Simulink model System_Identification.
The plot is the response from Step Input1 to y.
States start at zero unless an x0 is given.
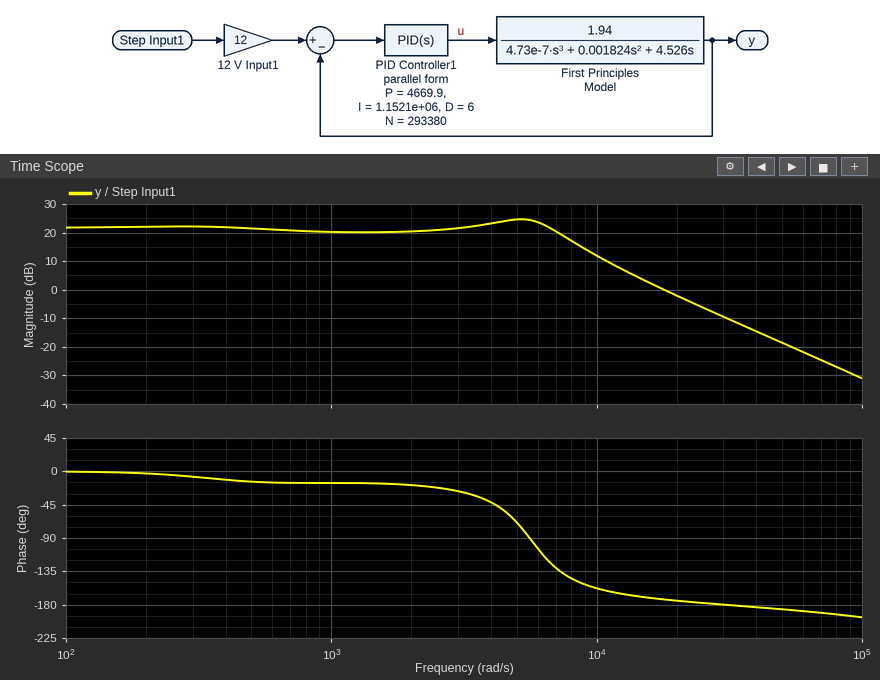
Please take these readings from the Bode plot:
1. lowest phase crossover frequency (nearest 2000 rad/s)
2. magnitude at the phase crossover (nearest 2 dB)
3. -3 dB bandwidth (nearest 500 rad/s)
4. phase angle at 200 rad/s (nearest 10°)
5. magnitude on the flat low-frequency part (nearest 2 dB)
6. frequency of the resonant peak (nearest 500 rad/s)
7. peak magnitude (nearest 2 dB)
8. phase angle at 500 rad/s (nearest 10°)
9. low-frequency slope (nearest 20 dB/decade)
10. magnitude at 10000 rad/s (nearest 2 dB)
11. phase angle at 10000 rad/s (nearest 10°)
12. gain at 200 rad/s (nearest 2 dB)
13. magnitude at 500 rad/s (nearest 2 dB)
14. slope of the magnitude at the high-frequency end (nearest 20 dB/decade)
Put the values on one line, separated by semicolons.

30000 rad/s; -10 dB; 7500 rad/s; 0°; 22 dB; 5000 rad/s; 24 dB; -10°; 0 dB/decade; 12 dB; -160°; 22 dB; 22 dB; -40 dB/decade
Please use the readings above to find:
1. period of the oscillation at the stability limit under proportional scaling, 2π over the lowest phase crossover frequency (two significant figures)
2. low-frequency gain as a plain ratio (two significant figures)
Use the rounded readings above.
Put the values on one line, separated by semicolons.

0.00021 s; 13
